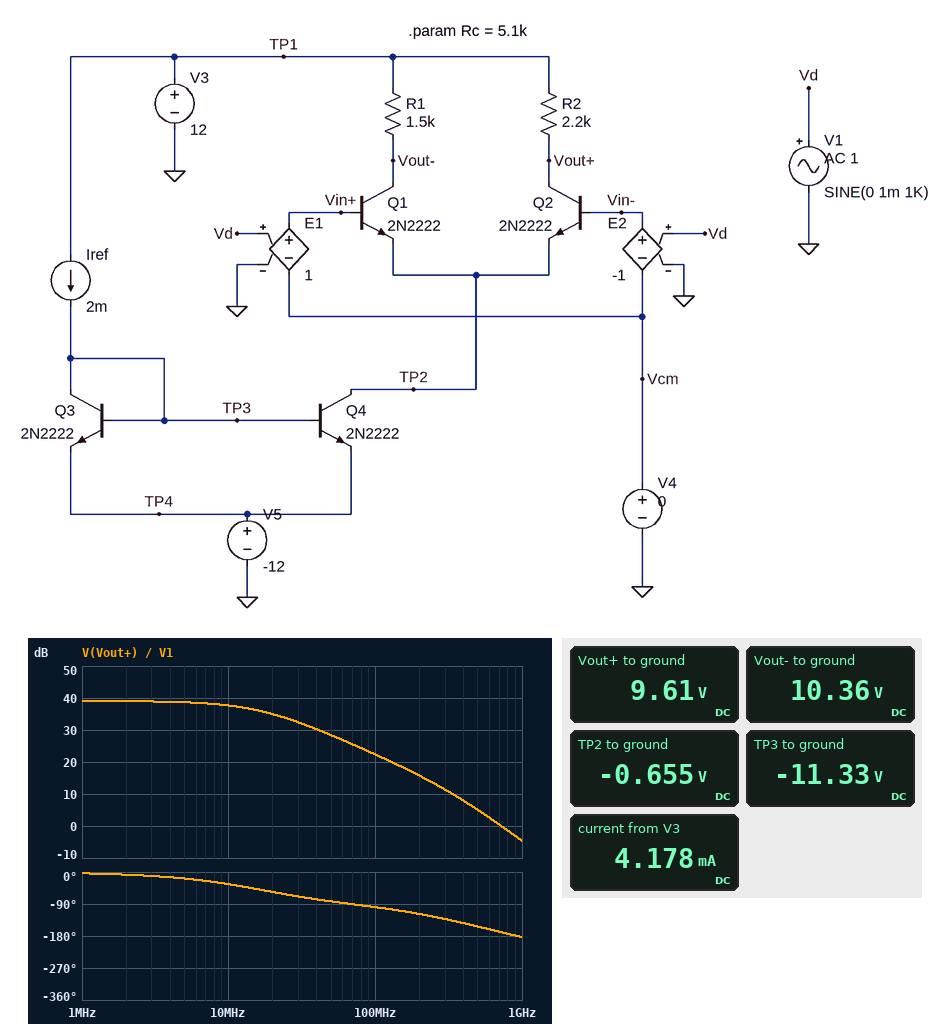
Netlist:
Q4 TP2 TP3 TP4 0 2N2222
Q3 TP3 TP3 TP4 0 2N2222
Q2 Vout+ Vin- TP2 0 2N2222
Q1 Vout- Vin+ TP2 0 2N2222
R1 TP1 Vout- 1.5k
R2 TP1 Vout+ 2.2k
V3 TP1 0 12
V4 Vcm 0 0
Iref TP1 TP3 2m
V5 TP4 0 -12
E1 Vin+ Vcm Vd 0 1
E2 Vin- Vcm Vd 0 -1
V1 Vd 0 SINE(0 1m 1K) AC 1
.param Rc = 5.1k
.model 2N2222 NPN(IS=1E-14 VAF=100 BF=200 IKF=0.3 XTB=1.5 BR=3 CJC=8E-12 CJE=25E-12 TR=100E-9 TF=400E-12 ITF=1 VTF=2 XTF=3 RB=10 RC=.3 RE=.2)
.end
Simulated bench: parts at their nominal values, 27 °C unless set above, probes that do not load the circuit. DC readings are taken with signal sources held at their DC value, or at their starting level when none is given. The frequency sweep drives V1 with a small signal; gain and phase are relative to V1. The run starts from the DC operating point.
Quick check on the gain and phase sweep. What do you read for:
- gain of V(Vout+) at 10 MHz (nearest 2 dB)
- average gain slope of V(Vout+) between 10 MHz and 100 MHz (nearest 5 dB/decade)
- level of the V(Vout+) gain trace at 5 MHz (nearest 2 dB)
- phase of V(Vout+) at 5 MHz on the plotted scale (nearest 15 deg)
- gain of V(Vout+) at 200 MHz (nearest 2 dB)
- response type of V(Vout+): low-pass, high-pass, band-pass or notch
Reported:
38 dB
-15 dB/decade
38 dB
-15 deg
16 dB
low-pass
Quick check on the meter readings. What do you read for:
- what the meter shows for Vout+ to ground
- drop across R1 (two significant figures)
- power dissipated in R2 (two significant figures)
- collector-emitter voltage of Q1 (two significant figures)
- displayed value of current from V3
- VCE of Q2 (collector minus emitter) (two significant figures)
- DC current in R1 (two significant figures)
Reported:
9.61 V
1.6 V
2.6 mW
11 V
4.178 mA
10 V
1.1 mA
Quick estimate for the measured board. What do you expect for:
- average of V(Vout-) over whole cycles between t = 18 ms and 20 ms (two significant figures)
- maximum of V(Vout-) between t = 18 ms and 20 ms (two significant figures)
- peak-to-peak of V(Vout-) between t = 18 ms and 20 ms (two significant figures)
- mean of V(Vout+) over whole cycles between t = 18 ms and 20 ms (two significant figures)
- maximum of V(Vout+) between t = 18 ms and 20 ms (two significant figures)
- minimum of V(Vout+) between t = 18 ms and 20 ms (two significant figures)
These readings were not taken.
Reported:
10 V
10 V
120 mV
9.6 V
9.7 V
9.5 V
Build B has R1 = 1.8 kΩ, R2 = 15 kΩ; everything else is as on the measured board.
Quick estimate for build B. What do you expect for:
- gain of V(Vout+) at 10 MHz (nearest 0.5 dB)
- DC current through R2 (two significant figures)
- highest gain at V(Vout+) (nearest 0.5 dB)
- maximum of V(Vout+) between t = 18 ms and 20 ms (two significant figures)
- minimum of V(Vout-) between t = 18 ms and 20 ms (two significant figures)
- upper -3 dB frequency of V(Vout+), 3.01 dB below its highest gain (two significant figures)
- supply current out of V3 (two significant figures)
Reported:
-1.0 dB
840 µA
14.0 dB
-610 mV
9.7 V
1.2 MHz
4.1 mA
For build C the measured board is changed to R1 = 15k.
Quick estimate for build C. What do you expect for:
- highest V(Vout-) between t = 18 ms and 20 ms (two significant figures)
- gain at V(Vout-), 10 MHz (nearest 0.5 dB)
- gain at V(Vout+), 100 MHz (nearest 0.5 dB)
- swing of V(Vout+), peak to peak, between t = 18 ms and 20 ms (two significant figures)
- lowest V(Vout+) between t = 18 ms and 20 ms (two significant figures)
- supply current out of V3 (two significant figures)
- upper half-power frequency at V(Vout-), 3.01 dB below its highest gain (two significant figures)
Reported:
-610 mV
-1.0 dB
23.0 dB
73 mV
9.2 V
4.1 mA
1.2 MHz
